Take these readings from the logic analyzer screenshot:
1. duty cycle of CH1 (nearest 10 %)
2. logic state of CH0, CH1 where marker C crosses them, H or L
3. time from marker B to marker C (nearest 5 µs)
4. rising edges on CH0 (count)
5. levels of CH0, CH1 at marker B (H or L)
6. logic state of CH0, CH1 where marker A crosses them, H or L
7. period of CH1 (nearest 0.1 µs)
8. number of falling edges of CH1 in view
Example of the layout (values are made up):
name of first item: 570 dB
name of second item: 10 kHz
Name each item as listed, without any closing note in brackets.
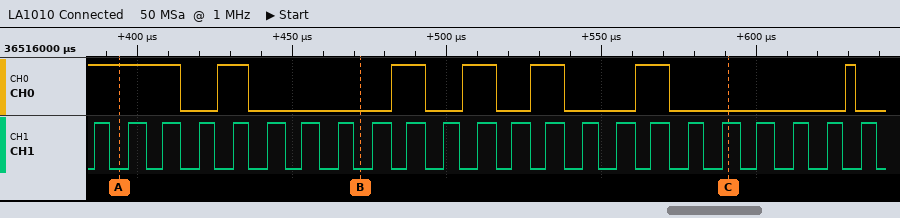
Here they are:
duty cycle of CH1: 50 %
logic state of CH0, CH1 where marker C crosses them, H or L: CH0=L, CH1=H
time from marker B to marker C: 120 µs
rising edges on CH0: 6
levels of CH0, CH1 at marker B: CH0=L, CH1=L
logic state of CH0, CH1 where marker A crosses them, H or L: CH0=H, CH1=L
period of CH1: 11.3 µs
number of falling edges of CH1 in view: 23
